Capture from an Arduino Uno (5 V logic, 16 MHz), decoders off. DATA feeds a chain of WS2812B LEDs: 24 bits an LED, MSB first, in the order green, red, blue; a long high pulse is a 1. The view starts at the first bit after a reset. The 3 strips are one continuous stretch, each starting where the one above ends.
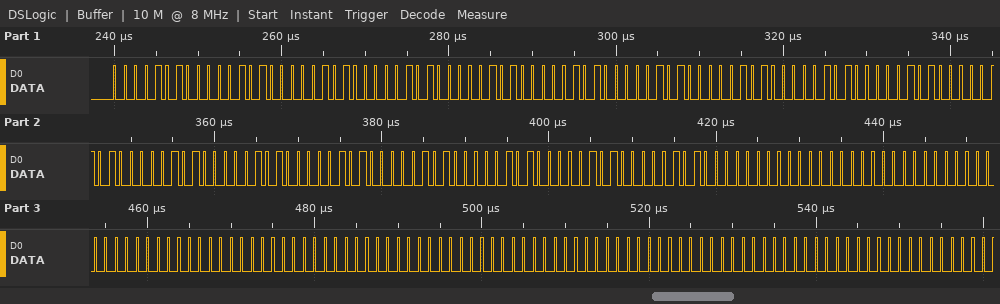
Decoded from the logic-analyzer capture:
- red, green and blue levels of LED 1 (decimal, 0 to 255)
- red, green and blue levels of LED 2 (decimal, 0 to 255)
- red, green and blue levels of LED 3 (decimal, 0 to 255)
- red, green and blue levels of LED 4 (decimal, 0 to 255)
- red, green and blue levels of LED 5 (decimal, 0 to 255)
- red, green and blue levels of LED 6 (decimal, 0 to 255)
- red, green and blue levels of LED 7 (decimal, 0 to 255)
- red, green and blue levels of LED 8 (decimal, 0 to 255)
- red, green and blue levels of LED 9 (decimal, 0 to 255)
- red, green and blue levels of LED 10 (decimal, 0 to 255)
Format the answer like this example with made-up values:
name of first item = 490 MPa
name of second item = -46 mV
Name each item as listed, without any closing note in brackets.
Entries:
red, green and blue levels of LED 1 = 10, 10, 10
red, green and blue levels of LED 2 = 10, 10, 10
red, green and blue levels of LED 3 = 10, 10, 10
red, green and blue levels of LED 4 = 10, 10, 10
red, green and blue levels of LED 5 = 10, 10, 10
red, green and blue levels of LED 6 = 10, 10, 10
red, green and blue levels of LED 7 = 0, 0, 0
red, green and blue levels of LED 8 = 0, 0, 0
red, green and blue levels of LED 9 = 0, 0, 0
red, green and blue levels of LED 10 = 0, 0, 0
